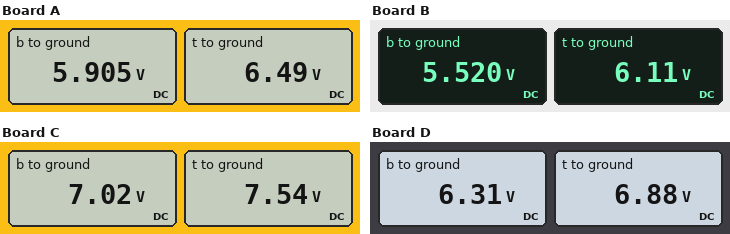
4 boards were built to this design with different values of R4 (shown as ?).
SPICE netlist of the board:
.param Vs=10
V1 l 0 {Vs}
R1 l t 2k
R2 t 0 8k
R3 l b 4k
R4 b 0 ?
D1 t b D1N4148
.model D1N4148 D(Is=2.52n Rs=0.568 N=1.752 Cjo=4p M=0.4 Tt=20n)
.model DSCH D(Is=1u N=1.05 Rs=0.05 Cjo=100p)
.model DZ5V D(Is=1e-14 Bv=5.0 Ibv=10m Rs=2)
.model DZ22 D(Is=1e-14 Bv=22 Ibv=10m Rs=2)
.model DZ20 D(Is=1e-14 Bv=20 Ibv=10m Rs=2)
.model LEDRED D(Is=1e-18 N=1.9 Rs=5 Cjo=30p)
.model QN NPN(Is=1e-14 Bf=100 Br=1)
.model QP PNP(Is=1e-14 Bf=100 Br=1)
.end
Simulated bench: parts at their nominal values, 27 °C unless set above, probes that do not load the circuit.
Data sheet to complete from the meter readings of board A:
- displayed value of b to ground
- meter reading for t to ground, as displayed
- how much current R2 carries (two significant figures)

5.905 V
6.49 V
810 µA
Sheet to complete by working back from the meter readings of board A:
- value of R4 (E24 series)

3 kΩ
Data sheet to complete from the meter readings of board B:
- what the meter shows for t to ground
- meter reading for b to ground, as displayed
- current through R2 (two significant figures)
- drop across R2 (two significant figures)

6.11 V
5.520 V
760 µA
6.1 V
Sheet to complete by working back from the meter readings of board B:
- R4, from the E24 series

2.4 kΩ
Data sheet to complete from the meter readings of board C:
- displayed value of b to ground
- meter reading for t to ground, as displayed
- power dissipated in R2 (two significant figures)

7.02 V
7.54 V
7.1 mW
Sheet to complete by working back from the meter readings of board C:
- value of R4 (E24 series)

6.8 kΩ
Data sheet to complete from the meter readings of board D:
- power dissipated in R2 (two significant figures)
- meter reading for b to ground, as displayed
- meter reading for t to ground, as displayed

5.9 mW
6.31 V
6.88 V
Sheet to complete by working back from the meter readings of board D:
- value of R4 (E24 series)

3.9 kΩ
